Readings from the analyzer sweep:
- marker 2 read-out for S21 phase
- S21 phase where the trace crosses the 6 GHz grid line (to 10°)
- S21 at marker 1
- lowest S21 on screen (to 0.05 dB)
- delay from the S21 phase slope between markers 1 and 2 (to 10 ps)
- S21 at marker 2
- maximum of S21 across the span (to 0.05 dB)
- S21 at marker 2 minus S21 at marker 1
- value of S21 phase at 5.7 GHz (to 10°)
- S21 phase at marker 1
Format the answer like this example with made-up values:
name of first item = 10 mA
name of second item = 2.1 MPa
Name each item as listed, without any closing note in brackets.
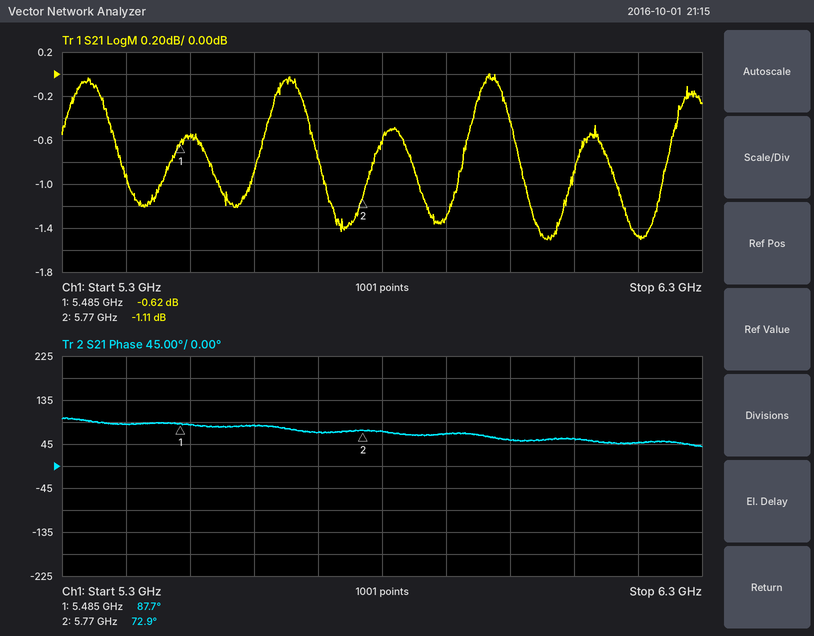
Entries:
marker 2 read-out for S21 phase = 72.9°
S21 phase where the trace crosses the 6 GHz grid line = 50°
S21 at marker 1 = -0.62 dB
lowest S21 on screen = -1.50 dB
delay from the S21 phase slope between markers 1 and 2 = 140 ps
S21 at marker 2 = -1.11 dB
maximum of S21 across the span = 0.00 dB
S21 at marker 2 minus S21 at marker 1 = -0.49 dB
value of S21 phase at 5.7 GHz = 70°
S21 phase at marker 1 = 87.7°
